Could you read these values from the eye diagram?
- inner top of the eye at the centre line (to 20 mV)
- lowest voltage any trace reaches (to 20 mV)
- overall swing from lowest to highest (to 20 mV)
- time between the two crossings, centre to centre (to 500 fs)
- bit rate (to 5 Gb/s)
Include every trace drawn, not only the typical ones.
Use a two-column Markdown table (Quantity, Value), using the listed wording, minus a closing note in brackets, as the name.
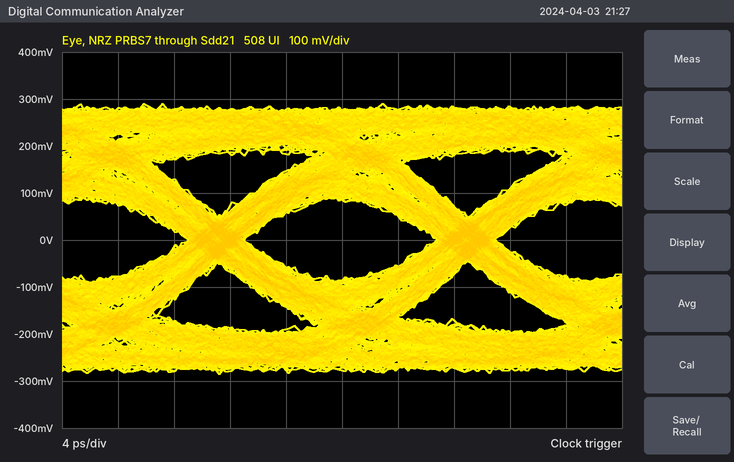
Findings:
| Quantity | Value |
|---|---|
| inner top of the eye at the centre line | 80 mV |
| lowest voltage any trace reaches | -280 mV |
| overall swing from lowest to highest | 580 mV |
| time between the two crossings, centre to centre | 18.0 ps |
| bit rate | 55 Gb/s |
